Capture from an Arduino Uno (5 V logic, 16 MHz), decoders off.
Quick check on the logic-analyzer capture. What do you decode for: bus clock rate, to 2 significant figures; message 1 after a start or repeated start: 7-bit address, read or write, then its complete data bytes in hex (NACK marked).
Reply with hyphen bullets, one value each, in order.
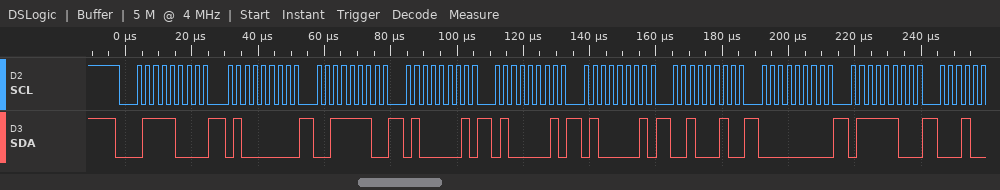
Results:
- 400 kHz
- 0x3C write: 40 3E 41 41 41 22 00 7C
